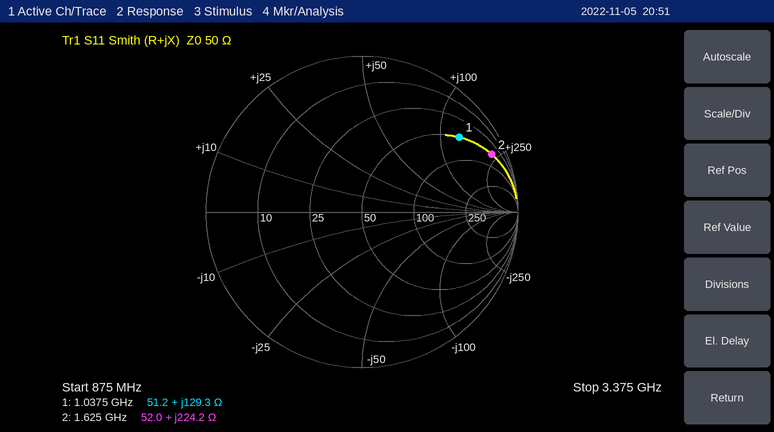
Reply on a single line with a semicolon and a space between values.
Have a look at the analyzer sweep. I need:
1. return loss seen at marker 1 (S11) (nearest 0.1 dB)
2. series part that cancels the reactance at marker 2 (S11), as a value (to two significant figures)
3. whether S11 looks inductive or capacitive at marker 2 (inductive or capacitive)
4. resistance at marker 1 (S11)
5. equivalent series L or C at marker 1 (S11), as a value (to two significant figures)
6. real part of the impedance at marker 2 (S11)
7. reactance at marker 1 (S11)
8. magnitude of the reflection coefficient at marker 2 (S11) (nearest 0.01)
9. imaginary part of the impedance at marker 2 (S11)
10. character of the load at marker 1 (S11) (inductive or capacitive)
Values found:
2.1 dB; 440 fF; inductive; 51.2 Ω; 20 nH; 52.0 Ω; +129.3 Ω; 0.91; +224.2 Ω; inductive
